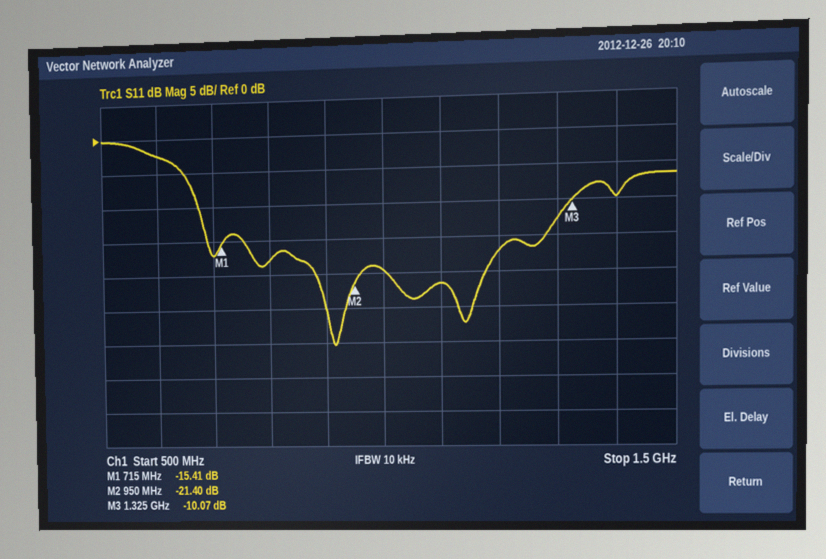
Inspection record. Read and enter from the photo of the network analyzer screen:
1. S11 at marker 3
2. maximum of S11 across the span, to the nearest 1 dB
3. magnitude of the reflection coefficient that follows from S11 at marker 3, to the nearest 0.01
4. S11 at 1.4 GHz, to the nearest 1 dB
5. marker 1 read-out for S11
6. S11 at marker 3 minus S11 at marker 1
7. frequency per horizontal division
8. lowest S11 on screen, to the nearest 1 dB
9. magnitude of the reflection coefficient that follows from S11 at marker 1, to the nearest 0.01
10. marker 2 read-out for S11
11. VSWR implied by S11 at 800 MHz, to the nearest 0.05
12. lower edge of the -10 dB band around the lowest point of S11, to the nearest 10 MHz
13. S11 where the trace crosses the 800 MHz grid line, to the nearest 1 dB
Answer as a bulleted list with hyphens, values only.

- -10.07 dB
- 0 dB
- 0.31
- -10 dB
- -15.41 dB
- 5.34 dB
- 100 MHz
- -30 dB
- 0.17
- -21.40 dB
- 1.30
- 670 MHz
- -18 dB
